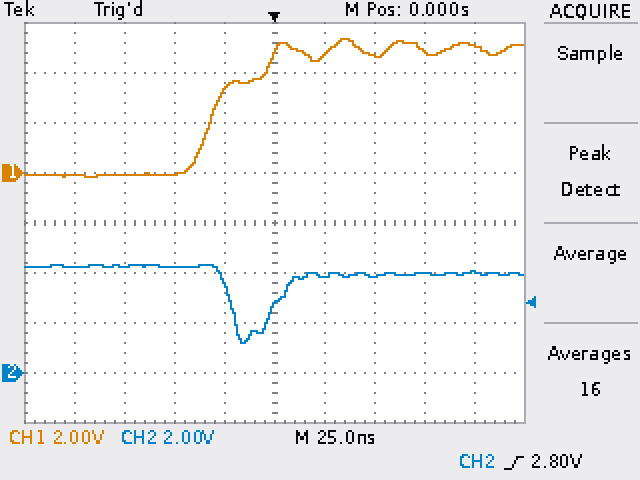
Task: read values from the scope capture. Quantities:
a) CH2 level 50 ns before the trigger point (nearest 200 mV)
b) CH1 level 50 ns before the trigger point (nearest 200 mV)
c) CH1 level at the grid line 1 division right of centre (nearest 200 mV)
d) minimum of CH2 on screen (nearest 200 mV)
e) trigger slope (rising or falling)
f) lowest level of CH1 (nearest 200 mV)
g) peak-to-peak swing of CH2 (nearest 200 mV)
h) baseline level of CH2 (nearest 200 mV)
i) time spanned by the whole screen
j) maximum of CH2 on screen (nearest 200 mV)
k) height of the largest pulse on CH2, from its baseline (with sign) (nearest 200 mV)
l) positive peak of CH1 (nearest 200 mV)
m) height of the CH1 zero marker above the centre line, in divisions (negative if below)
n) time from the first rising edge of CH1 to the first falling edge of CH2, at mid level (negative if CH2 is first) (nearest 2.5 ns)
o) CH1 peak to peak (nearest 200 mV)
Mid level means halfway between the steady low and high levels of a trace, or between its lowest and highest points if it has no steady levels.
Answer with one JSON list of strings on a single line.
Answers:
["4.2 V", "0.0 V", "4.8 V", "1.2 V", "rising", "-200 mV", "3.2 V", "4.0 V", "250 ns", "4.4 V", "-2.8 V", "5.4 V", "+1.0 div", "+7.5 ns", "5.6 V"]
